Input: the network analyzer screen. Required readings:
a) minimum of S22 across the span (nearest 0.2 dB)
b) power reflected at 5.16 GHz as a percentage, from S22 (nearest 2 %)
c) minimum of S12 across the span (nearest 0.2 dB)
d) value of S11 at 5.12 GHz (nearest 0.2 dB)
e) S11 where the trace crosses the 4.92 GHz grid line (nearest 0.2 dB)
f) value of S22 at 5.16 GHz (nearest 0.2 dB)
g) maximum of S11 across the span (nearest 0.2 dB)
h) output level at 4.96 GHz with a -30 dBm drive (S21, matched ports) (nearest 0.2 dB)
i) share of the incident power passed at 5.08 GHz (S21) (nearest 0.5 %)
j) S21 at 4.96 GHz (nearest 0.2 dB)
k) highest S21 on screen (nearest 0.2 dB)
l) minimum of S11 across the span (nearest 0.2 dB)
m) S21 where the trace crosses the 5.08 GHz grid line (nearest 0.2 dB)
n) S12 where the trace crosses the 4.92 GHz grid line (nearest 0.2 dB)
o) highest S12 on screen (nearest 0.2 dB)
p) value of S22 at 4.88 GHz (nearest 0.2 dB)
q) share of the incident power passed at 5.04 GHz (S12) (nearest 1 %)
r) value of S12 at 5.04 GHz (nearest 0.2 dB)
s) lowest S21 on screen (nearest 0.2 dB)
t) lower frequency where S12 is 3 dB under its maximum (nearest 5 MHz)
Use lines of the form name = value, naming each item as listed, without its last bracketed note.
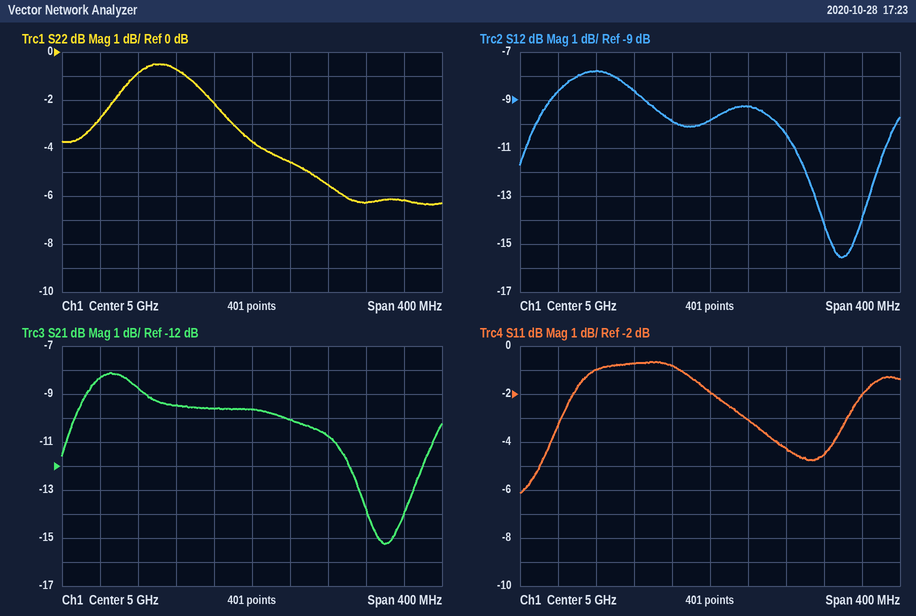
minimum of S22 across the span = -6.4 dB
power reflected at 5.16 GHz as a percentage, from S22 = 24 %
minimum of S12 across the span = -15.6 dB
value of S11 at 5.12 GHz = -4.6 dB
S11 where the trace crosses the 4.92 GHz grid line = -0.8 dB
value of S22 at 5.16 GHz = -6.2 dB
maximum of S11 across the span = -0.6 dB
output level at 4.96 GHz with a -30 dBm drive (S21, matched ports) = -39.6 dBm
share of the incident power passed at 5.08 GHz (S21) = 8.5 %
S21 at 4.96 GHz = -9.6 dB
highest S21 on screen = -8.2 dB
minimum of S11 across the span = -6.2 dB
S21 where the trace crosses the 5.08 GHz grid line = -10.8 dB
S12 where the trace crosses the 4.92 GHz grid line = -8.6 dB
highest S12 on screen = -7.8 dB
value of S22 at 4.88 GHz = -0.8 dB
share of the incident power passed at 5.04 GHz (S12) = 12 %
value of S12 at 5.04 GHz = -9.2 dB
lowest S21 on screen = -15.2 dB
lower frequency where S12 is 3 dB under its maximum = 4.810 GHz
